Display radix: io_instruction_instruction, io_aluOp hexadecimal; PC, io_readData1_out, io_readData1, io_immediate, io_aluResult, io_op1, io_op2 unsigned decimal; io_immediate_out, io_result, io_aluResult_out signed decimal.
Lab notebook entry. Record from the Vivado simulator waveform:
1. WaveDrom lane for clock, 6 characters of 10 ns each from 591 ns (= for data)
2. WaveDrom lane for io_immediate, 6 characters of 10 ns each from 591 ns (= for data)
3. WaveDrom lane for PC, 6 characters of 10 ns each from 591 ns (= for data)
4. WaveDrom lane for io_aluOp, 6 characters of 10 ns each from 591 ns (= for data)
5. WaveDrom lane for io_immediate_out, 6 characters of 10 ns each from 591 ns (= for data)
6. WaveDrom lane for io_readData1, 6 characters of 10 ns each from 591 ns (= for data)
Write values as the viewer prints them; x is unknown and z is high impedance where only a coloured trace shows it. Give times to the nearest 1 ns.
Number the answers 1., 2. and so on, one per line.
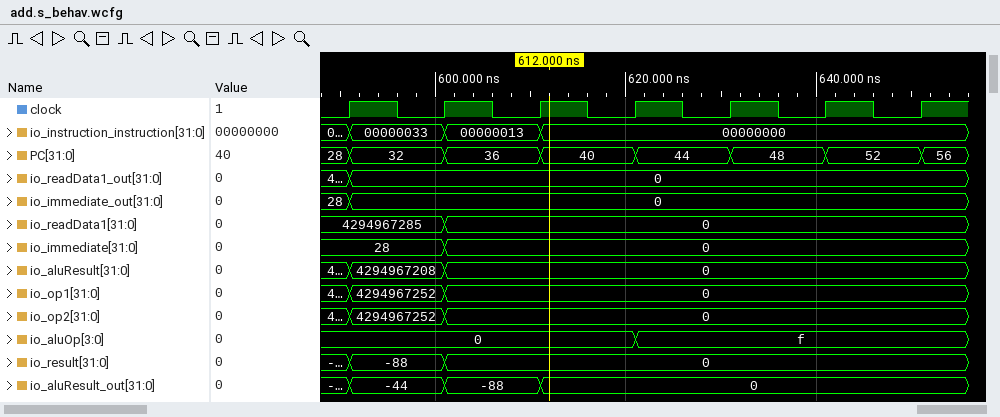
1. {name: 'clock', wave: 'p.....'}
2. {name: 'io_immediate', wave: '==....', data: '28 0'}
3. {name: 'PC', wave: '======', data: '32 36 40 44 48 52'}
4. {name: 'io_aluOp', wave: '=..=..', data: '0 f'}
5. {name: 'io_immediate_out', wave: '=.....', data: '0'}
6. {name: 'io_readData1', wave: '==....', data: '4294967285 0'}
